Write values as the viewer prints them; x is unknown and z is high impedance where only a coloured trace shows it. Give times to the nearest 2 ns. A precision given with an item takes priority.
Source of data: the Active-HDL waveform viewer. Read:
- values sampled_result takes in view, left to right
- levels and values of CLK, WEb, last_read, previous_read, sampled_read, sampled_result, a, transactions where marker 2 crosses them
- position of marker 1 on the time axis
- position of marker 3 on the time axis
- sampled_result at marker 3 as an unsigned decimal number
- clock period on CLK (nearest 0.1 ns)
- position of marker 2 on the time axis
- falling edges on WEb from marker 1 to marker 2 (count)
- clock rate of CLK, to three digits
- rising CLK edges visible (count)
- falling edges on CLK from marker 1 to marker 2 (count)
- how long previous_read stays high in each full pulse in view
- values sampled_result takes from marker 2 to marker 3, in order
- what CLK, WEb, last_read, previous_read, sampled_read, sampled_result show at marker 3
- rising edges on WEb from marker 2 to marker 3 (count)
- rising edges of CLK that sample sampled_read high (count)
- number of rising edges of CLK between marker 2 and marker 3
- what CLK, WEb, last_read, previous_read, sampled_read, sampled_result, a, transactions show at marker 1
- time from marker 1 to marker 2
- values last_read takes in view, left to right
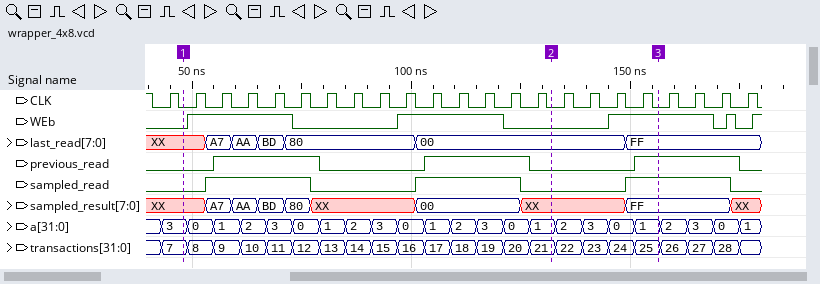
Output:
XX, A7, AA, BD, 80, XX, 00, XX, FF, XX
CLK=0, WEb=0, last_read=00, previous_read=0, sampled_read=0, sampled_result=XX, a=1, transactions=21
48 ns
156 ns
255
6 ns
132 ns
2
167 MHz
23
14
24 ns, 24 ns, 24 ns
XX, FF
CLK=0, WEb=1, last_read=FF, previous_read=1, sampled_read=1, sampled_result=FF
1
12
4
CLK=0, WEb=0, last_read=XX, previous_read=0, sampled_read=0, sampled_result=XX, a=3, transactions=7
84 ns
XX, A7, AA, BD, 80, 00, FF
